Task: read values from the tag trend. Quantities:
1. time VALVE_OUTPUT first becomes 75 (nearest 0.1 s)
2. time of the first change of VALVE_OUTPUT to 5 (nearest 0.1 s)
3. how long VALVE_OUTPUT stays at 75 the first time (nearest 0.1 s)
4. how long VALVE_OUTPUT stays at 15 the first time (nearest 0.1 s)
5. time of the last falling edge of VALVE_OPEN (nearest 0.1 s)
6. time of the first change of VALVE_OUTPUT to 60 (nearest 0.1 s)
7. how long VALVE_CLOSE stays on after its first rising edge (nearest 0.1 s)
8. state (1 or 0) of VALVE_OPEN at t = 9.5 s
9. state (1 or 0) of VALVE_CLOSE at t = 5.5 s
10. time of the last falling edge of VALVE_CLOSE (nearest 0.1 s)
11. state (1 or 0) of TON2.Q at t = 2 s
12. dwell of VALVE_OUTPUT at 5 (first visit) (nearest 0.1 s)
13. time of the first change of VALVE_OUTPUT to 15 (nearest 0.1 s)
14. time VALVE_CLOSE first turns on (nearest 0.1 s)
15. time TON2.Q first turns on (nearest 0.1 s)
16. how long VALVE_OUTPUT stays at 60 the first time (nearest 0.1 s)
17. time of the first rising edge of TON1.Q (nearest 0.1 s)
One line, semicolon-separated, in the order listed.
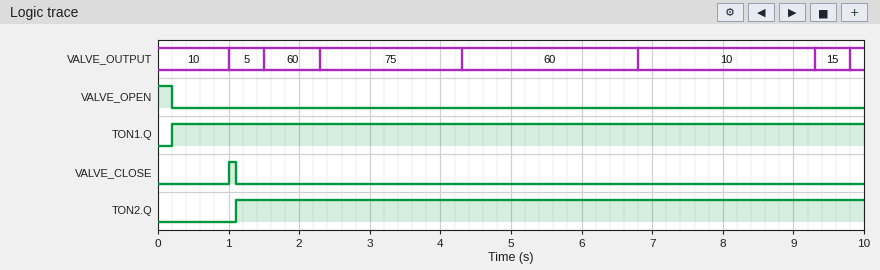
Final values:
2.3 s; 1.0 s; 2.0 s; 0.5 s; 0.2 s; 1.5 s; 0.1 s; 0; 0; 1.1 s; 1; 0.5 s; 9.3 s; 1.0 s; 1.1 s; 0.8 s; 0.2 s
